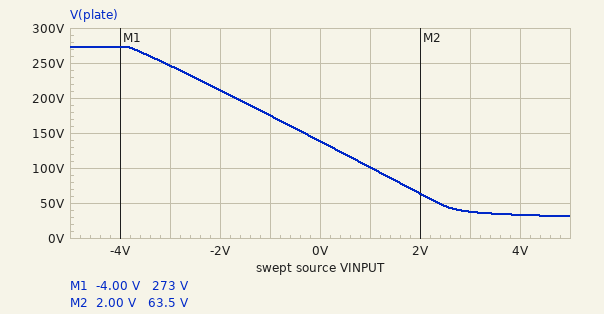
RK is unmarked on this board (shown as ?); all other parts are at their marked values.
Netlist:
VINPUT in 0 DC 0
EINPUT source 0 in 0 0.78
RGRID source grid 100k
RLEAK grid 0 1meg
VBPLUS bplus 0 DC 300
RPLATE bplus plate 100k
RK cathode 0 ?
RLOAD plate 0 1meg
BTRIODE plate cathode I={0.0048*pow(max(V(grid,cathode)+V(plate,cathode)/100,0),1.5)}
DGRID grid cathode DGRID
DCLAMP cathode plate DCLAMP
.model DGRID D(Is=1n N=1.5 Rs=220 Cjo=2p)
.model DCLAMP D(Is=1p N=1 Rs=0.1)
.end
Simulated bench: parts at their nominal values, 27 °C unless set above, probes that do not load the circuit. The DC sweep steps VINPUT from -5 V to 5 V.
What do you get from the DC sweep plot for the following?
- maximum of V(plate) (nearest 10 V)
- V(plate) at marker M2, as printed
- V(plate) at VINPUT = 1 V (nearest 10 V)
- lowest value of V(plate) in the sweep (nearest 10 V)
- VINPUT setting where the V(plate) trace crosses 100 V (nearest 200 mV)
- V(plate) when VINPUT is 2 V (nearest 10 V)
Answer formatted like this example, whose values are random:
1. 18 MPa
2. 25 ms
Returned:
1. 270 V
2. 63.5 V
3. 100 V
4. 30 V
5. 1.0 V
6. 60 V
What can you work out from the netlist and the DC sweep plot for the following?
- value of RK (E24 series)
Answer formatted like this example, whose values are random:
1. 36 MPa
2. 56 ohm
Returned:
1. 620 Ω
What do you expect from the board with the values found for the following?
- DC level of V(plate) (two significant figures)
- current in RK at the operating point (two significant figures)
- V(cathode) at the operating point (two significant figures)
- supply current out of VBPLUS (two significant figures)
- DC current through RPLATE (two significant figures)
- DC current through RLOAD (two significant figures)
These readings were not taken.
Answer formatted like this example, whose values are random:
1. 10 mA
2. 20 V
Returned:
1. 140 V
2. 1.5 mA
3. 920 mV
4. 1.6 mA
5. 1.6 mA
6. 140 µA
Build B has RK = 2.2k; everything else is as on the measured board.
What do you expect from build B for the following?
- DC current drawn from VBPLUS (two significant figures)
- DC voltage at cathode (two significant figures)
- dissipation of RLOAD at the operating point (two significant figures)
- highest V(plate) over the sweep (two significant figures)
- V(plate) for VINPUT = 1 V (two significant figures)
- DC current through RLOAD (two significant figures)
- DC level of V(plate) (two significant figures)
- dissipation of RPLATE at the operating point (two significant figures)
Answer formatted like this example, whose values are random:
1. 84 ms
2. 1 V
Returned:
1. 980 µA
2. 1.7 V
3. 41 mW
4. 270 V
5. 180 V
6. 200 µA
7. 200 V
8. 96 mW
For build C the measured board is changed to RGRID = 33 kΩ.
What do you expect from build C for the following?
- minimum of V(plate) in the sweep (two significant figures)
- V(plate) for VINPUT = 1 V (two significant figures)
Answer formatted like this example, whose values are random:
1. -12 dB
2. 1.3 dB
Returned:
1. 27 V
2. 99 V
